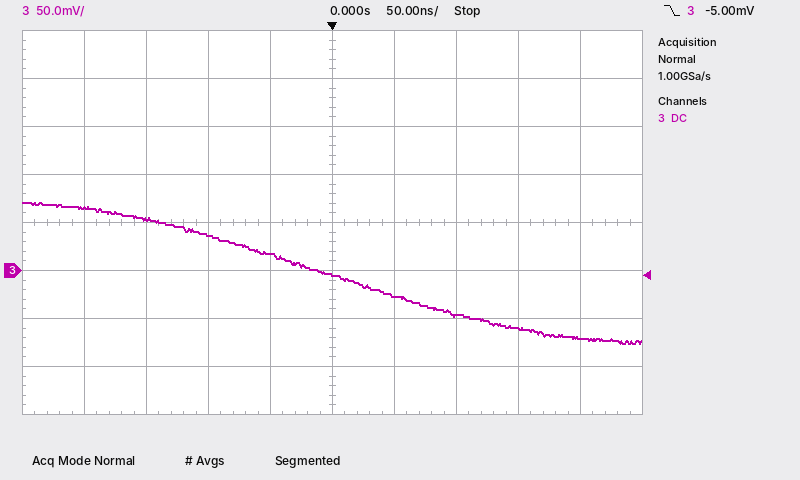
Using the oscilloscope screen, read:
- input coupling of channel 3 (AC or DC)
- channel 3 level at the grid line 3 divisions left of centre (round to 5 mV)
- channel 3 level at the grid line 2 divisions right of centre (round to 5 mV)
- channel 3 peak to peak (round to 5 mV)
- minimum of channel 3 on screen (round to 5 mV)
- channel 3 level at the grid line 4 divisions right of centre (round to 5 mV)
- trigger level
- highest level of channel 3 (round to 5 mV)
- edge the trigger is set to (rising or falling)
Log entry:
DC
55 mV
-45 mV
145 mV
-75 mV
-70 mV
-5.00 mV
70 mV
falling
